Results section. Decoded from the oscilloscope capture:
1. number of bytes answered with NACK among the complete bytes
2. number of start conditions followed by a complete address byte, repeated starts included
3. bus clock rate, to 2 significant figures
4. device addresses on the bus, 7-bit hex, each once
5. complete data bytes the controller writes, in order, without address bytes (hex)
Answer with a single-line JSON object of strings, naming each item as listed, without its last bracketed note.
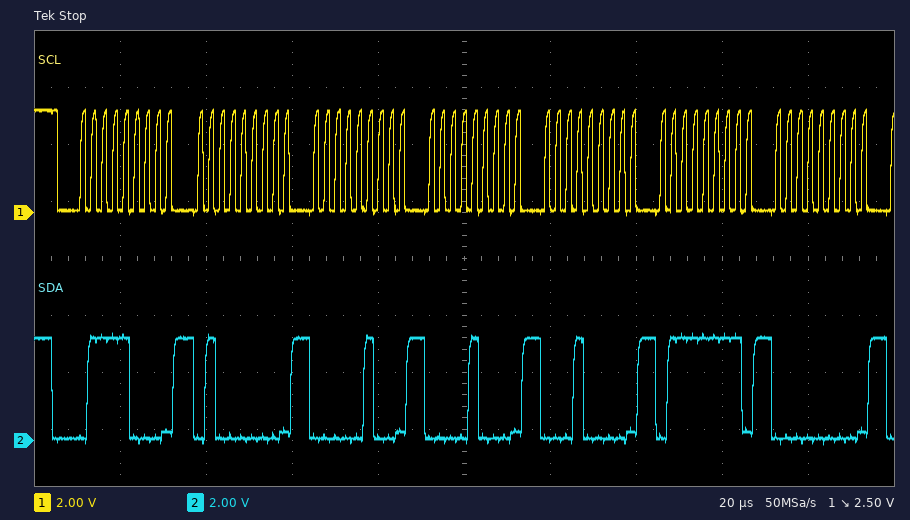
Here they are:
{"number of bytes answered with NACK among the complete bytes": "0", "number of start conditions followed by a complete address byte, repeated starts included": "1", "bus clock rate, to 2 significant figures": "400 kHz", "device addresses on the bus, 7-bit hex, each once": "0x3C", "complete data bytes the controller writes, in order, without address bytes": "40 04 08 10 7F 00"}
